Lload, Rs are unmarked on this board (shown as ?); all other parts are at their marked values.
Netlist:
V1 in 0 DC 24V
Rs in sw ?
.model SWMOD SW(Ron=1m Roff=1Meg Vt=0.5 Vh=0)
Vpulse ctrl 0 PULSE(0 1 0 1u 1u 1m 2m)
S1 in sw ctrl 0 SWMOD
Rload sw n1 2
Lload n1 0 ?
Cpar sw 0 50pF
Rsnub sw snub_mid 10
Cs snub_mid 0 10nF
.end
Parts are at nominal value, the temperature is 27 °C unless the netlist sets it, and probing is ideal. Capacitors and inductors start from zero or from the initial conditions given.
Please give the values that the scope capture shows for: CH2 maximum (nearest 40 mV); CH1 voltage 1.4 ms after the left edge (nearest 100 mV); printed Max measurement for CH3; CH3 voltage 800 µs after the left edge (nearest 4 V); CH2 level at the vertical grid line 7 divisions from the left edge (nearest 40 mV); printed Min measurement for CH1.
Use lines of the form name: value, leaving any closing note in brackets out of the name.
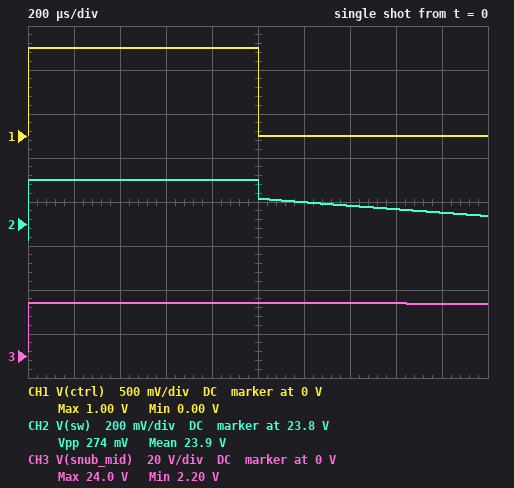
CH2 maximum: 24.00 V
CH1 voltage 1.4 ms after the left edge: 0 V
printed Max measurement for CH3: 24.0 V
CH3 voltage 800 µs after the left edge: 24 V
CH2 level at the vertical grid line 7 divisions from the left edge: 23.88 V
printed Min measurement for CH1: 0.00 V
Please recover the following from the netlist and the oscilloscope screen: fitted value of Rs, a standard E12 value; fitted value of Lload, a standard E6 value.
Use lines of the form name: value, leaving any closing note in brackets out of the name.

fitted value of Rs, a standard E12 value: 0.12 Ω
fitted value of Lload, a standard E6 value: 33 mH
